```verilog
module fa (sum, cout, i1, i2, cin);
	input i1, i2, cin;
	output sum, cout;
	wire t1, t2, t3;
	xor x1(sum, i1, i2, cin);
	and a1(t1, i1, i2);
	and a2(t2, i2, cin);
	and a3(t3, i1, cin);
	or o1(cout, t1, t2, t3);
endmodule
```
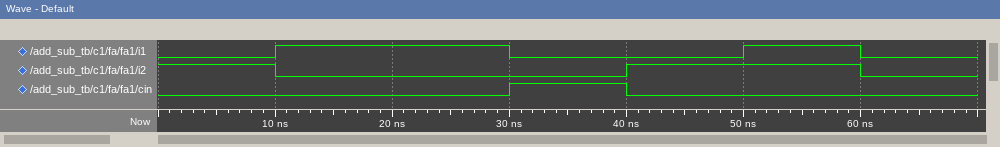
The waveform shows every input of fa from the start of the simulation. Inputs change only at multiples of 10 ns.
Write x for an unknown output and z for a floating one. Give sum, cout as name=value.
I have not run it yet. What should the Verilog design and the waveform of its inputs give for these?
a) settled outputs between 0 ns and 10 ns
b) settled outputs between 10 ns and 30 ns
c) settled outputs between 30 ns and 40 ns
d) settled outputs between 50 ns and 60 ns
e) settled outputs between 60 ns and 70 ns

sum=1, cout=0
sum=1, cout=0
sum=1, cout=0
sum=0, cout=1
sum=0, cout=0
